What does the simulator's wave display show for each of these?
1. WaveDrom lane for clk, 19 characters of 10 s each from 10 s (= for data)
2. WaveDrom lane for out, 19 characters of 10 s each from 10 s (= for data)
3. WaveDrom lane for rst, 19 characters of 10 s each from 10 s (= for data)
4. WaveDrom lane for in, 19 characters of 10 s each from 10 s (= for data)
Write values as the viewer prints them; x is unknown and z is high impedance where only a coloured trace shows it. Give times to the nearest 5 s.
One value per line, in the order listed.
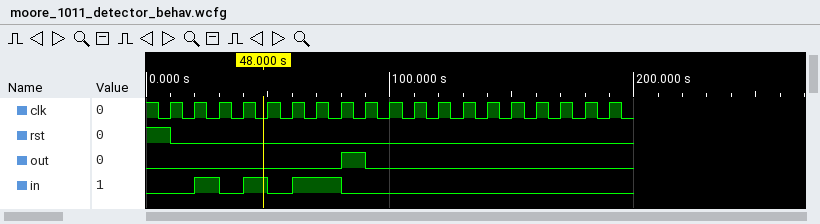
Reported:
{name: 'clk', wave: 'p..................'}
{name: 'out', wave: '0......10..........'}
{name: 'rst', wave: '0..................'}
{name: 'in', wave: '010101.0...........'}
